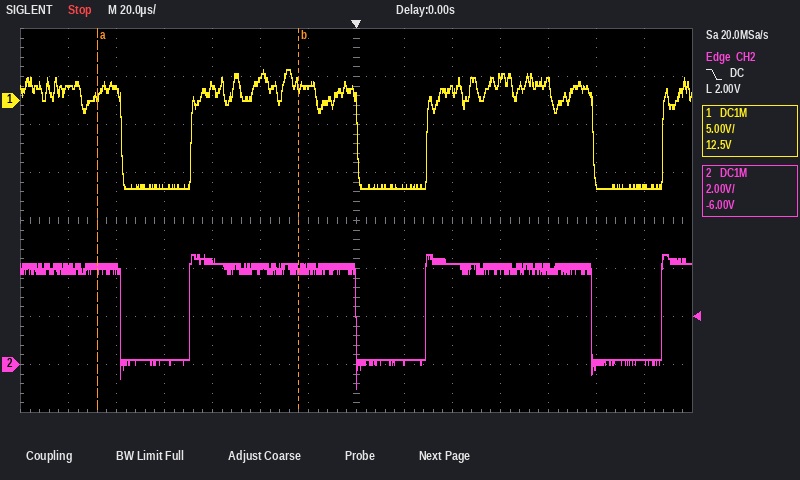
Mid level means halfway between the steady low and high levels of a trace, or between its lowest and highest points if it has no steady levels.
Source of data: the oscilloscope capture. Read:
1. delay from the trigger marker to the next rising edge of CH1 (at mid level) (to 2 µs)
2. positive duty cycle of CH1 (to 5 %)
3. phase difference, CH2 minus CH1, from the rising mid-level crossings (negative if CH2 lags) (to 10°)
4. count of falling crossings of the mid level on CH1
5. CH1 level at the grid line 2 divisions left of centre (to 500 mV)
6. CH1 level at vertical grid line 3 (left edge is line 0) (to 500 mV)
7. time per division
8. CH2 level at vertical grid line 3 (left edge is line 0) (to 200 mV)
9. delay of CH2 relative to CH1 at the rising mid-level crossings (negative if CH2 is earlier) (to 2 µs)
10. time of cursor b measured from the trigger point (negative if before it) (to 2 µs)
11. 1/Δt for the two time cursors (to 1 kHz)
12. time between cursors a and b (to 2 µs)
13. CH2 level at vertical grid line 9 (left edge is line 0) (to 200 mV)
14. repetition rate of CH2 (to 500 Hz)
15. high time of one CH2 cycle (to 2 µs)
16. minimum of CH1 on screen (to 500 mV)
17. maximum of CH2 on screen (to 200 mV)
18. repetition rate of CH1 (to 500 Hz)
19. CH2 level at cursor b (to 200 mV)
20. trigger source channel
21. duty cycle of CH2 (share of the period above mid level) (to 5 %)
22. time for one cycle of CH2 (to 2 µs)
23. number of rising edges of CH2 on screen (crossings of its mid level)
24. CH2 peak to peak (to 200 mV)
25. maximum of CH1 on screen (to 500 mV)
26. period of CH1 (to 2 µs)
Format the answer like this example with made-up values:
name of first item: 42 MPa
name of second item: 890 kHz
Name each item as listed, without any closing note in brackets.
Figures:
delay from the trigger marker to the next rising edge of CH1 (at mid level): 30 µs
positive duty cycle of CH1: 70 %
phase difference, CH2 minus CH1, from the rising mid-level crossings (negative if CH2 lags): 0°
count of falling crossings of the mid level on CH1: 3
CH1 level at the grid line 2 divisions left of centre: 2.5 V
CH1 level at vertical grid line 3 (left edge is line 0): -9.0 V
time per division: 20 µs
CH2 level at vertical grid line 3 (left edge is line 0): 200 mV
delay of CH2 relative to CH1 at the rising mid-level crossings (negative if CH2 is earlier): 0 µs
time of cursor b measured from the trigger point (negative if before it): -24 µs
1/Δt for the two time cursors: 12 kHz
time between cursors a and b: 84 µs
CH2 level at vertical grid line 9 (left edge is line 0): 4.2 V
repetition rate of CH2: 10.0 kHz
high time of one CH2 cycle: 70 µs
minimum of CH1 on screen: -9.0 V
maximum of CH2 on screen: 4.6 V
repetition rate of CH1: 10.0 kHz
CH2 level at cursor b: 4.0 V
trigger source channel: CH2
duty cycle of CH2 (share of the period above mid level): 70 %
time for one cycle of CH2: 98 µs
number of rising edges of CH2 on screen: 3
CH2 peak to peak: 5.6 V
maximum of CH1 on screen: 3.0 V
period of CH1: 98 µs
